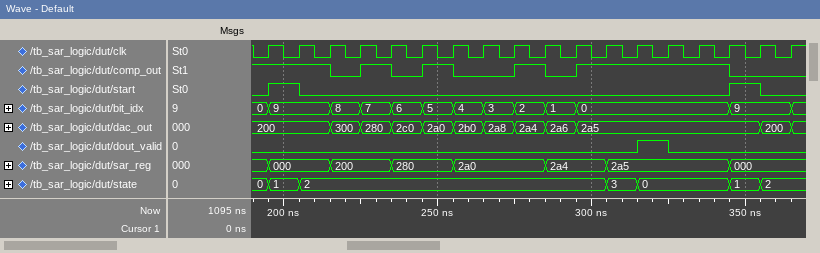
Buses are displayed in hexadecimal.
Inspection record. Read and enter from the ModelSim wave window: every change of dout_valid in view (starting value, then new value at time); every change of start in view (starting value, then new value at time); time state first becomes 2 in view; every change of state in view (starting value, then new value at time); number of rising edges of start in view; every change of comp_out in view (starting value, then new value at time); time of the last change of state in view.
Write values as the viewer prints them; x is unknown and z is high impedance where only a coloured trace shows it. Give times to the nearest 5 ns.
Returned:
0, 1 at 315 ns, 0 at 325 ns
0, 1 at 195 ns, 0 at 205 ns, 1 at 345 ns, 0 at 355 ns
205 ns
0, 1 at 195 ns, 2 at 205 ns, 3 at 305 ns, 0 at 315 ns, 1 at 345 ns, 2 at 355 ns
2
1, 0 at 215 ns, 1 at 225 ns, 0 at 235 ns, 1 at 245 ns, 0 at 255 ns, 1 at 275 ns, 0 at 285 ns, 1 at 295 ns, 0 at 345 ns
355 ns
